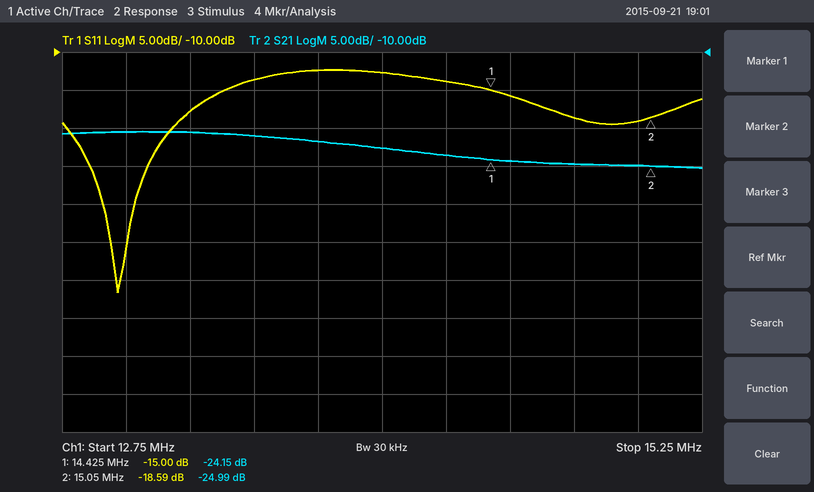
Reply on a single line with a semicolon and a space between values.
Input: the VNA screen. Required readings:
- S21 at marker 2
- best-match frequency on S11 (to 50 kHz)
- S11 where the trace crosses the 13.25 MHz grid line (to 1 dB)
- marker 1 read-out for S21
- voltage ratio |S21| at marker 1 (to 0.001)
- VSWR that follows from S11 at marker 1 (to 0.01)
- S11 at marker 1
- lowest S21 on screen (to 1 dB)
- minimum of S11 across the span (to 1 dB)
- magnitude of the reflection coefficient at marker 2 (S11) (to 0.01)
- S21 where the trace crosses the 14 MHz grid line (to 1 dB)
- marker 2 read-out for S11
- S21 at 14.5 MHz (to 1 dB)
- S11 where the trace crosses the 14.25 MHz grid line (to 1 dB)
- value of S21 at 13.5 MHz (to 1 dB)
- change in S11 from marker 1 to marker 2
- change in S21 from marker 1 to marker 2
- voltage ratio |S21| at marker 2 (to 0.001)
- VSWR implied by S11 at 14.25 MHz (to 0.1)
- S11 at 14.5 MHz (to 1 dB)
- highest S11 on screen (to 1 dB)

-24.99 dB; 12.95 MHz; -18 dB; -24.15 dB; 0.062; 1.43; -15.00 dB; -25 dB; -42 dB; 0.12; -23 dB; -18.59 dB; -24 dB; -14 dB; -21 dB; -3.59 dB; -0.84 dB; 0.056; 1.5; -16 dB; -12 dB
